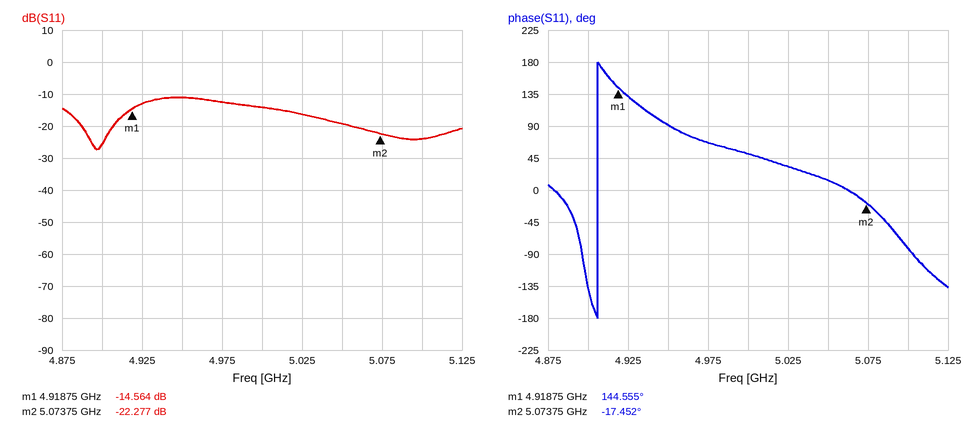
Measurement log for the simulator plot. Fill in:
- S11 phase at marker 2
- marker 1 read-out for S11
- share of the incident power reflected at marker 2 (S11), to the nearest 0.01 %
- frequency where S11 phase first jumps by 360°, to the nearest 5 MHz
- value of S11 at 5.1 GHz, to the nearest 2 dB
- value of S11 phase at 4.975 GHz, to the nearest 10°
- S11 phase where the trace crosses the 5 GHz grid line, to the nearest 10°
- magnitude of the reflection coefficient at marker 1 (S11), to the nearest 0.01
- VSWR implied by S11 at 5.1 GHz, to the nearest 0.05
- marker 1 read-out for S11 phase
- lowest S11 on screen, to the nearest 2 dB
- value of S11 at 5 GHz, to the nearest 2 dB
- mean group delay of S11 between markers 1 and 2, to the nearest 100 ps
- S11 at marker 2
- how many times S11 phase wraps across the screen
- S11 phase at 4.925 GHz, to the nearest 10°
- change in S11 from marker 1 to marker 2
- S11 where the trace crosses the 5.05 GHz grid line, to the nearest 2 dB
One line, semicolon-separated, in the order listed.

-17.452°; -14.564 dB; 0.59 %; 4.905 GHz; -24 dB; 70°; 50°; 0.19; 1.15; 144.555°; -28 dB; -14 dB; 2.9 ns; -22.277 dB; 1; 130°; -7.713 dB; -20 dB
